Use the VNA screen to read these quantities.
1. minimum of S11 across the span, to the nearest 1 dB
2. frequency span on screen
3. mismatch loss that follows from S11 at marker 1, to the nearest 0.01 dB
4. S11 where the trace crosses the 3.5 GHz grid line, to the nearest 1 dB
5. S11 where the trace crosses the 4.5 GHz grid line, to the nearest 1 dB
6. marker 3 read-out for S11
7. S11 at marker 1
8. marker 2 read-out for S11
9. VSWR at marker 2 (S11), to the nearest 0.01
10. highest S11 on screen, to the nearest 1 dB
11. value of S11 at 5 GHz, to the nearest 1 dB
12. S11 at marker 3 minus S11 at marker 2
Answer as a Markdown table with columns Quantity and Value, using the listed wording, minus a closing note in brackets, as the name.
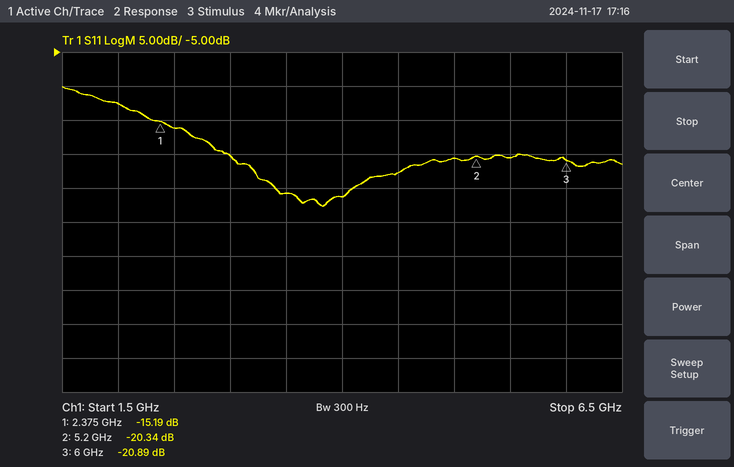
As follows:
| Quantity | Value |
|---|---|
| minimum of S11 across the span, to the nearest 1 dB | -28 dB |
| frequency span on screen | 5 GHz |
| mismatch loss that follows from S11 at marker 1, to the nearest 0.01 dB | 0.13 dB |
| S11 where the trace crosses the 3.5 GHz grid line, to the nearest 1 dB | -26 dB |
| S11 where the trace crosses the 4.5 GHz grid line, to the nearest 1 dB | -23 dB |
| marker 3 read-out for S11 | -20.89 dB |
| S11 at marker 1 | -15.19 dB |
| marker 2 read-out for S11 | -20.34 dB |
| VSWR at marker 2 (S11), to the nearest 0.01 | 1.21 |
| highest S11 on screen, to the nearest 1 dB | -10 dB |
| value of S11 at 5 GHz, to the nearest 1 dB | -21 dB |
| S11 at marker 3 minus S11 at marker 2 | -0.55 dB |
